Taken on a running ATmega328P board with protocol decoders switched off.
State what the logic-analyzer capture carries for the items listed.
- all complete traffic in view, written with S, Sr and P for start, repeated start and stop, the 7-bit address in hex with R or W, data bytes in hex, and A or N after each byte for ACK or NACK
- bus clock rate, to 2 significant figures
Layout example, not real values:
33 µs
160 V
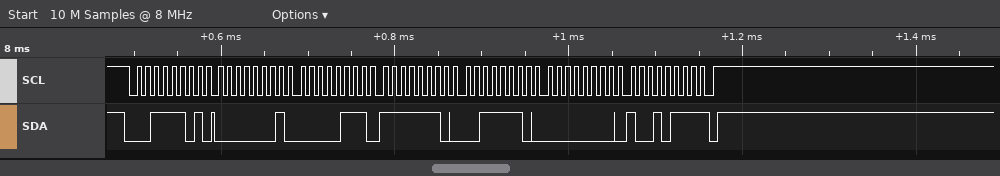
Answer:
S 1ER A 01 A 07 A FE A 3E A 00 A 97 N P
100 kHz
